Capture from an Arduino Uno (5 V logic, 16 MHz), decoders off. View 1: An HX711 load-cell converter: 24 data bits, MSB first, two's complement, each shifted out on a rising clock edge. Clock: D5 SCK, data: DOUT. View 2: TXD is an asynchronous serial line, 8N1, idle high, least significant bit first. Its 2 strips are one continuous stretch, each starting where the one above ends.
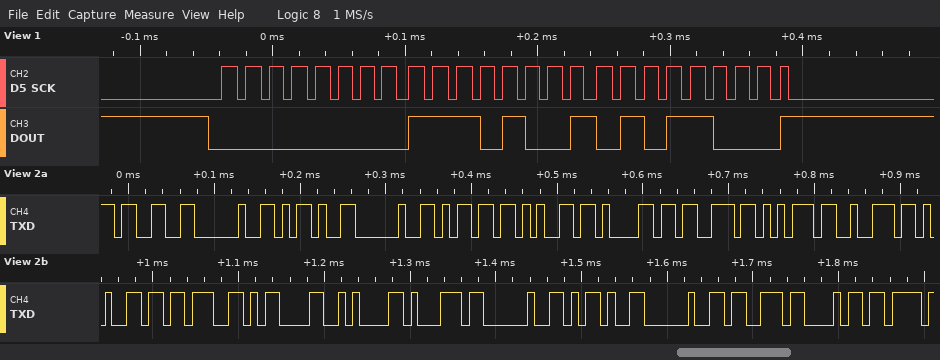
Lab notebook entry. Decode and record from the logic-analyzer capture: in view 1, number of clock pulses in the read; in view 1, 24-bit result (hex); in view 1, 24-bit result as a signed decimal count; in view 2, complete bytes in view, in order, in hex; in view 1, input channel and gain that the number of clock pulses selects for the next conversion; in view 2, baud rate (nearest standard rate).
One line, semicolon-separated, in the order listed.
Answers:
25; 0x00E958; 59736; 0x33 0x20 0x2D 0x20 0x6D 0x65 0x61 0x73 0x75 0x72 0x65 0x3B 0x0D 0x0A 0x71 0x20 0x2D 0x20 0x73 0x68; channel A, gain 128; 115200 baud
